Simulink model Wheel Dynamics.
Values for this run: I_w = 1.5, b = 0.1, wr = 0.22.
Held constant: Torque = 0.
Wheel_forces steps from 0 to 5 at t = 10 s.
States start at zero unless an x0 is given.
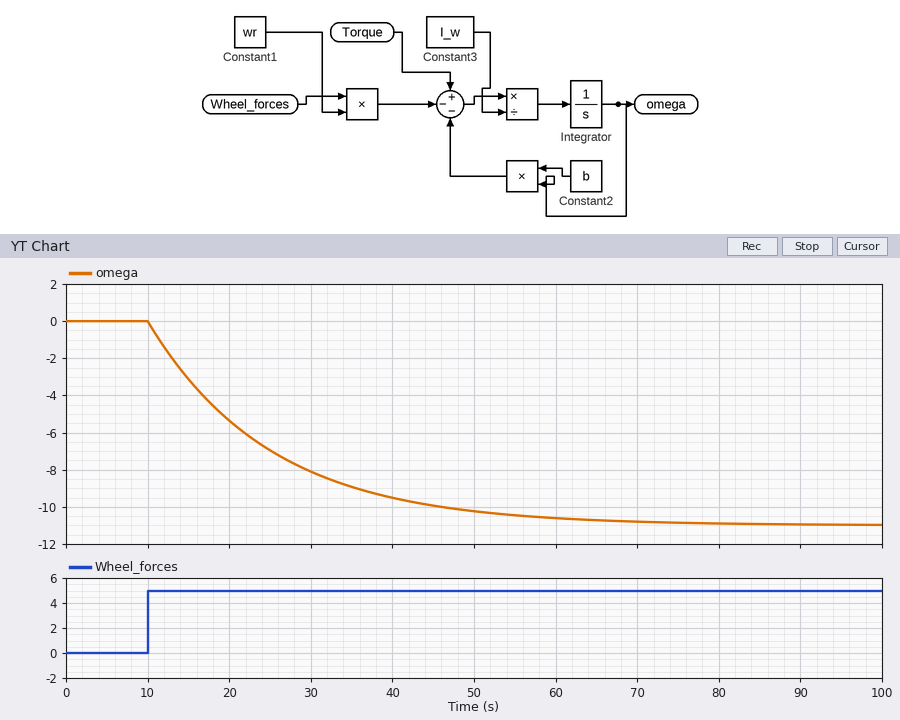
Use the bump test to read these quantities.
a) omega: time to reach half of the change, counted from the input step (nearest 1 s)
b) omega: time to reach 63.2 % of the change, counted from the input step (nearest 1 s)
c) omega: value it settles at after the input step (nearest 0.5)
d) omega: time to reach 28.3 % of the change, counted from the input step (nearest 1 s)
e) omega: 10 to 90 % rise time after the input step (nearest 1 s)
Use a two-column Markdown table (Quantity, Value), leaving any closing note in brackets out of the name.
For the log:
| Quantity | Value |
|---|---|
| omega: time to reach half of the change, counted from the input step | 10 s |
| omega: time to reach 63.2 % of the change, counted from the input step | 15 s |
| omega: value it settles at after the input step | -11.0 |
| omega: time to reach 28.3 % of the change, counted from the input step | 5 s |
| omega: 10 to 90 % rise time after the input step | 33 s |
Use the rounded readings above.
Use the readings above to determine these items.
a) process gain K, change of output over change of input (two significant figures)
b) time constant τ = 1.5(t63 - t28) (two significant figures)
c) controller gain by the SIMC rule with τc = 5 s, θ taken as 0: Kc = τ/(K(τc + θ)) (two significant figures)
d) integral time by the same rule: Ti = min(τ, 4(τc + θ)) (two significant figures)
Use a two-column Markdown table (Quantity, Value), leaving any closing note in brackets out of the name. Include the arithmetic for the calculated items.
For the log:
| Quantity | Value |
|---|---|
| process gain K, change of output over change of input | (-11 - 0) / 5 = -2.2 |
| time constant τ = 1.5(t63 - t28) | 1.5 × (15 - 5) = 15 s |
| controller gain by the SIMC rule with τc = 5 s, θ taken as 0: Kc = τ/(K(τc + θ)) | 15 / (-2.2 × (5 + 0)) = -1.4 |
| integral time by the same rule: Ti = min(τ, 4(τc + θ)) | min(15, 4 × (5 + 0)) = 15 s |
